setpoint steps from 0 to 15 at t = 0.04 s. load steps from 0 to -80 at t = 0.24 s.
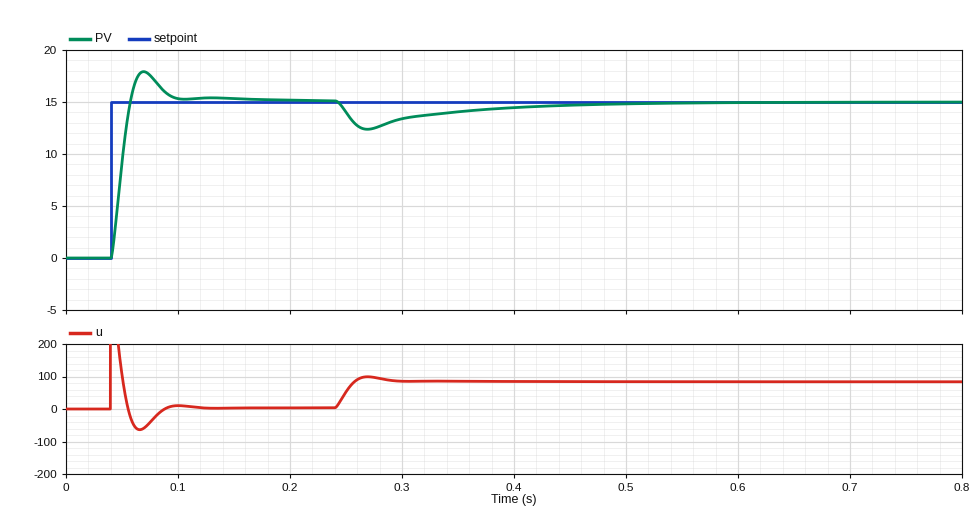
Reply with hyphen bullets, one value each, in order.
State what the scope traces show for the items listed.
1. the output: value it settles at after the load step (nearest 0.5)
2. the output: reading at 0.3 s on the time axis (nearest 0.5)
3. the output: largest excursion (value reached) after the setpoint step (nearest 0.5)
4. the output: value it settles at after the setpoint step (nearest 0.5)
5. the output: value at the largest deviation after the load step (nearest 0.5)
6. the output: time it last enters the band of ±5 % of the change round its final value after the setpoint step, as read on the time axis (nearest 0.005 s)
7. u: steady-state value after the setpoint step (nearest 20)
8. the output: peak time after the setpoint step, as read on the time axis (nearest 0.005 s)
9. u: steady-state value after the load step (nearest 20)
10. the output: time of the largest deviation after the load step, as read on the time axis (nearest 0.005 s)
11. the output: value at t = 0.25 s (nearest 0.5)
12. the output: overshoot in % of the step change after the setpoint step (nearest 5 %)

- 15.0
- 13.5
- 18.0
- 15.0
- 12.5
- 0.090 s
- 0
- 0.070 s
- 80
- 0.270 s
- 14.0
- 20 %
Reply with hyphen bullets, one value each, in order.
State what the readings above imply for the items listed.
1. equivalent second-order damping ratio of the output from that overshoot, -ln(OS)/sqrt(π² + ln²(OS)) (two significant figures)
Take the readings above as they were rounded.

- 0.46
